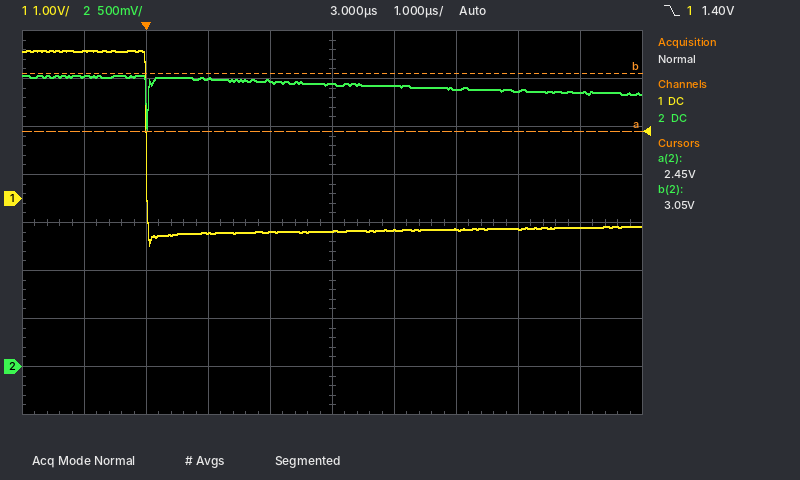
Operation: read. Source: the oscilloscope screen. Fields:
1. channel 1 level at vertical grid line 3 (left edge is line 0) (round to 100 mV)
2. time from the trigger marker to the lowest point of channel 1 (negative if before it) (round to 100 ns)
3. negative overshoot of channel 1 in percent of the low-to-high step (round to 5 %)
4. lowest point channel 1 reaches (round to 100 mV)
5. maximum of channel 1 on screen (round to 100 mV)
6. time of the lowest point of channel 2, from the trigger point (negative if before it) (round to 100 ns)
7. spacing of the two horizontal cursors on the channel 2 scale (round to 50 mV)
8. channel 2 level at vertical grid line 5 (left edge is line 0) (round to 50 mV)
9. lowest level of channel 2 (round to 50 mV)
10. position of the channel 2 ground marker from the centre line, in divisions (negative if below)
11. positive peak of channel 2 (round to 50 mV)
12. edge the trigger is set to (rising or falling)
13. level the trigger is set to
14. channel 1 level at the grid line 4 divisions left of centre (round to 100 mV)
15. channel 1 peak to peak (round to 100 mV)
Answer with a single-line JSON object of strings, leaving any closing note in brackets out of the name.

{"channel 1 level at vertical grid line 3 (left edge is line 0)": "-700 mV", "time from the trigger marker to the lowest point of channel 1 (negative if before it)": "+100 ns", "negative overshoot of channel 1 in percent of the low-to-high step": "10 %", "lowest point channel 1 reaches": "-1.0 V", "maximum of channel 1 on screen": "3.1 V", "time of the lowest point of channel 2, from the trigger point (negative if before it)": "0.0 µs", "spacing of the two horizontal cursors on the channel 2 scale": "600 mV", "channel 2 level at vertical grid line 5 (left edge is line 0)": "2.95 V", "lowest level of channel 2": "2.45 V", "position of the channel 2 ground marker from the centre line, in divisions": "-3.0 div", "positive peak of channel 2": "3.05 V", "edge the trigger is set to": "falling", "level the trigger is set to": "1.40 V", "channel 1 level at the grid line 4 divisions left of centre": "3.1 V", "channel 1 peak to peak": "4.1 V"}
